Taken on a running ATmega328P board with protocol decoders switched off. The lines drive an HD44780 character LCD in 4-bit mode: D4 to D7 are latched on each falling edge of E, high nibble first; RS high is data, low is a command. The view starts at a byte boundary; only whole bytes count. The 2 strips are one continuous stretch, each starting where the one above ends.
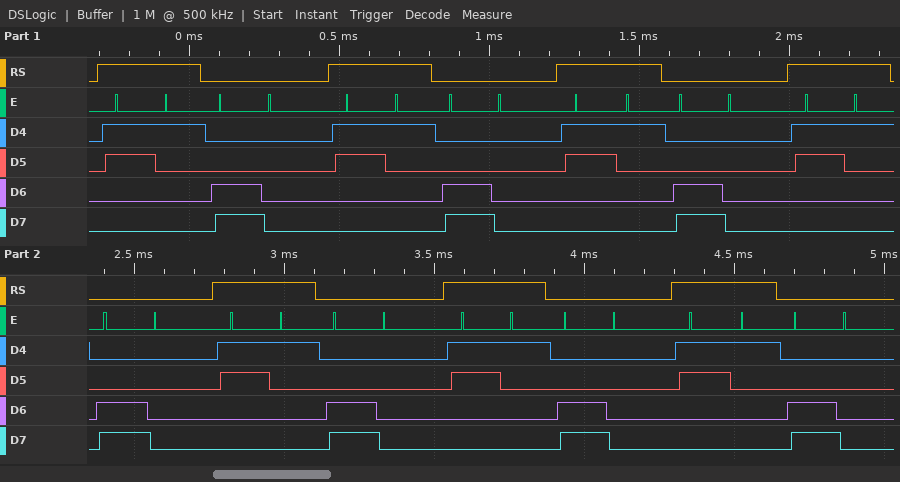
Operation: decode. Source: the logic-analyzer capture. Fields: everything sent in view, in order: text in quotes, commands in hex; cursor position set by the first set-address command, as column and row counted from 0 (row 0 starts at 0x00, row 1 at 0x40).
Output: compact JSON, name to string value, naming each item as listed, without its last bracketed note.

{"everything sent in view, in order: text in quotes, commands in hex": "\"1\" 0xC0 \"1\" 0xC0 \"1\" 0xC0 \"1\" 0xC0 \"1\" 0xC0 \"1\" 0xC0 \"1\" 0xC0", "cursor position set by the first set-address command, as column and row counted from 0": "column 0, row 1"}
